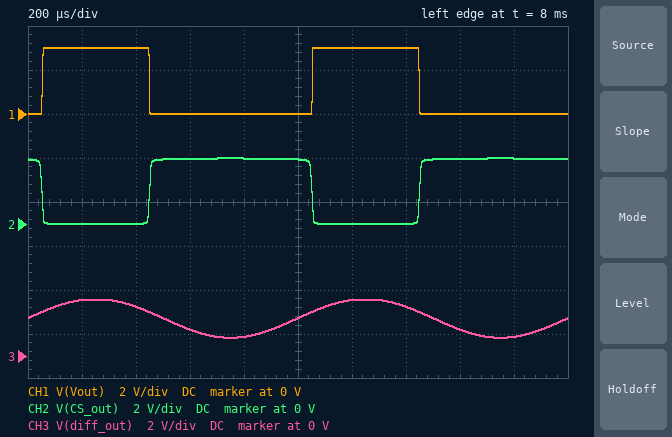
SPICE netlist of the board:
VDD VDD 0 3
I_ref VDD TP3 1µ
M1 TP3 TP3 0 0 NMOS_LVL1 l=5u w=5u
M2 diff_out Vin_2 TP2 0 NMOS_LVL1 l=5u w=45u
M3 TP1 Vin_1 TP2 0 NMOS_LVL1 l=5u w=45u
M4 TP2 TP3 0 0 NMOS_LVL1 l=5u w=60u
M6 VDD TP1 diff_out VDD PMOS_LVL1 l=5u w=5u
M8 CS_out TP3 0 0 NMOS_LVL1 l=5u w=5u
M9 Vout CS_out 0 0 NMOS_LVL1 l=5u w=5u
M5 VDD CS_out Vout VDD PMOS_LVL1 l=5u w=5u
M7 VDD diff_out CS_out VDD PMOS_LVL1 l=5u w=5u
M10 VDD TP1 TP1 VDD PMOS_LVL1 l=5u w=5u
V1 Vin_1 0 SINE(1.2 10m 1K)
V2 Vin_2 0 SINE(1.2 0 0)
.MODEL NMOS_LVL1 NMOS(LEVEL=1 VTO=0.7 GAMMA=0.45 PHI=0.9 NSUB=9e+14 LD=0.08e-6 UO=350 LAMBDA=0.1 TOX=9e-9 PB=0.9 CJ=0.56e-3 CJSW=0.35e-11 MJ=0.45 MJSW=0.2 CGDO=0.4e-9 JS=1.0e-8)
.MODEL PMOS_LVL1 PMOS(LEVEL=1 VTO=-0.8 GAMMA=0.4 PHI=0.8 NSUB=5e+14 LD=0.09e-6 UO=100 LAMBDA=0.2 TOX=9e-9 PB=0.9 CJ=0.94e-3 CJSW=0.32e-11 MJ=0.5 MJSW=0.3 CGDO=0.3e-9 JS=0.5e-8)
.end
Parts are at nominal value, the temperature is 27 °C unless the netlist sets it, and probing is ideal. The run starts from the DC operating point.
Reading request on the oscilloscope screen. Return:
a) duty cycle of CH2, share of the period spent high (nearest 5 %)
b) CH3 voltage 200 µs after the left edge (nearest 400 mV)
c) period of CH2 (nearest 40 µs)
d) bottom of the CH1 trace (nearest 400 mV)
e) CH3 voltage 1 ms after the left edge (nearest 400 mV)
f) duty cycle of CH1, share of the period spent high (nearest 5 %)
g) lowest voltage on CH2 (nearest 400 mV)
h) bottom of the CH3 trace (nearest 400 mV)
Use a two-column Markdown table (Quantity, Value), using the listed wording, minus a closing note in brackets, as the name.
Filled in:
| Quantity | Value |
|---|---|
| duty cycle of CH2, share of the period spent high | 60 % |
| CH3 voltage 200 µs after the left edge | 2.4 V |
| period of CH2 | 1.00 ms |
| bottom of the CH1 trace | 0 V |
| CH3 voltage 1 ms after the left edge | 1.6 V |
| duty cycle of CH1, share of the period spent high | 40 % |
| lowest voltage on CH2 | 0 V |
| bottom of the CH3 trace | 800 mV |
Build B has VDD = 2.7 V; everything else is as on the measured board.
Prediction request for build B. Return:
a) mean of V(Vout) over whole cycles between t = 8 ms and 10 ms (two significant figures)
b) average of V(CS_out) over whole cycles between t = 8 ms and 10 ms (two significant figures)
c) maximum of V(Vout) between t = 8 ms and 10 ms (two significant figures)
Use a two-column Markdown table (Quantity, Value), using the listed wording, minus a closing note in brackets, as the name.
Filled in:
| Quantity | Value |
|---|---|
| mean of V(Vout) over whole cycles between t = 8 ms and 10 ms | 1.1 V |
| average of V(CS_out) over whole cycles between t = 8 ms and 10 ms | 1.6 V |
| maximum of V(Vout) between t = 8 ms and 10 ms | 2.7 V |
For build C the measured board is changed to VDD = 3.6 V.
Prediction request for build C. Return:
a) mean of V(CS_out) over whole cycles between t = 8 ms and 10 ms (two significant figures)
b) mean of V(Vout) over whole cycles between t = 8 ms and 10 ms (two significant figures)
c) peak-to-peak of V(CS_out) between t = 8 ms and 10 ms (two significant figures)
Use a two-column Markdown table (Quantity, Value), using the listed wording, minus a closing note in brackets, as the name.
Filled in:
| Quantity | Value |
|---|---|
| mean of V(CS_out) over whole cycles between t = 8 ms and 10 ms | 2.1 V |
| mean of V(Vout) over whole cycles between t = 8 ms and 10 ms | 1.4 V |
| peak-to-peak of V(CS_out) between t = 8 ms and 10 ms | 3.6 V |
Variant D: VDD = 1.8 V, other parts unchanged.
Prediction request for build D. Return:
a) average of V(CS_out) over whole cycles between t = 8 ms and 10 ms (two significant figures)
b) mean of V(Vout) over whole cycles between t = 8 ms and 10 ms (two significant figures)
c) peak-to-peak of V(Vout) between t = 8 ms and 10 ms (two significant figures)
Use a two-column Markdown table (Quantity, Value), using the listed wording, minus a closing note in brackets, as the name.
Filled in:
| Quantity | Value |
|---|---|
| average of V(CS_out) over whole cycles between t = 8 ms and 10 ms | 1.1 V |
| mean of V(Vout) over whole cycles between t = 8 ms and 10 ms | 700 mV |
| peak-to-peak of V(Vout) between t = 8 ms and 10 ms | 1.8 V |
